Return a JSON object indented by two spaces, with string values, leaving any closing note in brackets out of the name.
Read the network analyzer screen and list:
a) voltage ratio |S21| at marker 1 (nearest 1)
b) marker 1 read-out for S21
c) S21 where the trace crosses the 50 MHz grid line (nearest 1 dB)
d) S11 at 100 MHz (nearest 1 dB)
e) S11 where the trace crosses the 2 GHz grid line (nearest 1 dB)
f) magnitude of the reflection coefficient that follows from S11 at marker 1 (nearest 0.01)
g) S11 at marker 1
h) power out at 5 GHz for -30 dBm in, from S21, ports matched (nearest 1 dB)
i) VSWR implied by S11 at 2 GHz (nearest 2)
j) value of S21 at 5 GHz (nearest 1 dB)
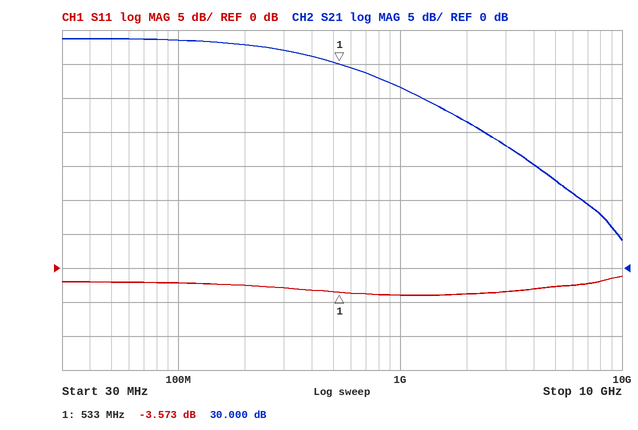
{
  "voltage ratio |S21| at marker 1": "32",
  "marker 1 read-out for S21": "30.000 dB",
  "S21 where the trace crosses the 50 MHz grid line": "34 dB",
  "S11 at 100 MHz": "-2 dB",
  "S11 where the trace crosses the 2 GHz grid line": "-4 dB",
  "magnitude of the reflection coefficient that follows from S11 at marker 1": "0.66",
  "S11 at marker 1": "-3.573 dB",
  "power out at 5 GHz for -30 dBm in, from S21, ports matched": "-17 dBm",
  "VSWR implied by S11 at 2 GHz": "4",
  "value of S21 at 5 GHz": "13 dB"
}
